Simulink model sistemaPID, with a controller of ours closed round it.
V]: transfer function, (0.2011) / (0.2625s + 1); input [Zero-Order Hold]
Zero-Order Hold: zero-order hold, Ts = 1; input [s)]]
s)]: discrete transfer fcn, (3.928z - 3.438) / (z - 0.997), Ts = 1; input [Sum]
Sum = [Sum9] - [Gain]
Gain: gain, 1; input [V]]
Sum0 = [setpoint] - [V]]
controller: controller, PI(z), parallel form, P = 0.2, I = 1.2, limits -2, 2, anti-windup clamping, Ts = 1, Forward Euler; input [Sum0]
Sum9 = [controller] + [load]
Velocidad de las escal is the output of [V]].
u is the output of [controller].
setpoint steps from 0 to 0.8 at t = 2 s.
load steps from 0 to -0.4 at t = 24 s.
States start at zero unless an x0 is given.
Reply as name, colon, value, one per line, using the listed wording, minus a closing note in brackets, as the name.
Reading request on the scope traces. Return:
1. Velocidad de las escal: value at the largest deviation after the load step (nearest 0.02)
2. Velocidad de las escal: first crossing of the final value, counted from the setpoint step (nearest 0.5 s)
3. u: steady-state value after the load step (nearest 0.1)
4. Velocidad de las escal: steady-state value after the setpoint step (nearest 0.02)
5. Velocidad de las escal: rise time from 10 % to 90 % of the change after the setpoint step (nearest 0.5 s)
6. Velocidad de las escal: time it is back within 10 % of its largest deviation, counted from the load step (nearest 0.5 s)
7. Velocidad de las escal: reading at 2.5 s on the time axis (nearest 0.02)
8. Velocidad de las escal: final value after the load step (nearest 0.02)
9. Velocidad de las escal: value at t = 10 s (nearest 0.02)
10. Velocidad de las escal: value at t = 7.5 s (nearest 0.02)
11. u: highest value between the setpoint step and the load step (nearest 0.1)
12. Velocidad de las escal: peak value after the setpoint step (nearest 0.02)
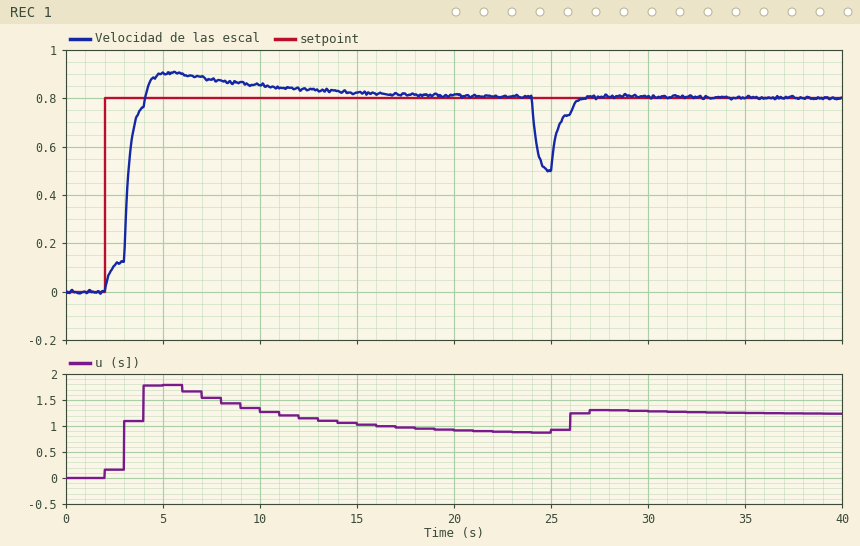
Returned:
Velocidad de las escal: value at the largest deviation after the load step: 0.50
Velocidad de las escal: first crossing of the final value, counted from the setpoint step: 2.0 s
u: steady-state value after the load step: 1.2
Velocidad de las escal: steady-state value after the setpoint step: 0.80
Velocidad de las escal: rise time from 10 % to 90 % of the change after the setpoint step: 1.5 s
Velocidad de las escal: time it is back within 10 % of its largest deviation, counted from the load step: 2.0 s
Velocidad de las escal: reading at 2.5 s on the time axis: 0.10
Velocidad de las escal: final value after the load step: 0.80
Velocidad de las escal: value at t = 10 s: 0.86
Velocidad de las escal: value at t = 7.5 s: 0.88
u: highest value between the setpoint step and the load step: 1.8
Velocidad de las escal: peak value after the setpoint step: 0.90
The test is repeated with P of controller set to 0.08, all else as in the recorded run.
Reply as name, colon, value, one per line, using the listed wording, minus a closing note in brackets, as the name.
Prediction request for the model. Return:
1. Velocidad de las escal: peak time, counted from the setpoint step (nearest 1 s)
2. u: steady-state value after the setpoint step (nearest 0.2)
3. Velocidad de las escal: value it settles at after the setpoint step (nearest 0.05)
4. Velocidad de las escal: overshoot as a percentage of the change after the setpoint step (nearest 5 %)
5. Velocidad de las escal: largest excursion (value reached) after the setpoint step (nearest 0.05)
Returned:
Velocidad de las escal: peak time, counted from the setpoint step: 3 s
u: steady-state value after the setpoint step: 0.8
Velocidad de las escal: value it settles at after the setpoint step: 0.80
Velocidad de las escal: overshoot as a percentage of the change after the setpoint step: 20 %
Velocidad de las escal: largest excursion (value reached) after the setpoint step: 0.95
